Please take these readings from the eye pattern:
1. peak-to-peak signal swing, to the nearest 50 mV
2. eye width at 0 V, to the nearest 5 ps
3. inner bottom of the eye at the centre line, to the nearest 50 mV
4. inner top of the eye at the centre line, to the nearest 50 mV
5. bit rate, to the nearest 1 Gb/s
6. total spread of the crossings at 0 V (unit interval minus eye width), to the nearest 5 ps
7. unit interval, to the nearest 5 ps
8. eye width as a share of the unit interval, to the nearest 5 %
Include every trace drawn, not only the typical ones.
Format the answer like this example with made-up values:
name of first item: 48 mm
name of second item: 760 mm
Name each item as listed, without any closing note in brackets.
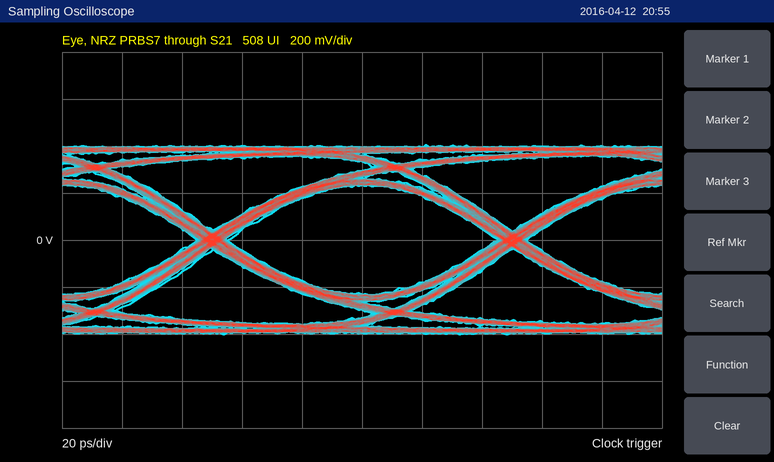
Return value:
peak-to-peak signal swing, to the nearest 50 mV: 800 mV
eye width at 0 V, to the nearest 5 ps: 90 ps
inner bottom of the eye at the centre line, to the nearest 50 mV: -250 mV
inner top of the eye at the centre line, to the nearest 50 mV: 250 mV
bit rate, to the nearest 1 Gb/s: 10 Gb/s
total spread of the crossings at 0 V (unit interval minus eye width), to the nearest 5 ps: 10 ps
unit interval, to the nearest 5 ps: 100 ps
eye width as a share of the unit interval, to the nearest 5 %: 90 %
